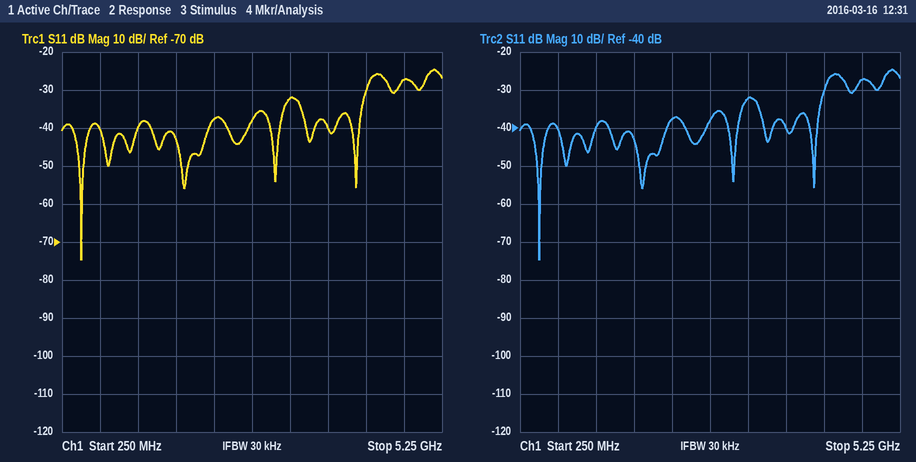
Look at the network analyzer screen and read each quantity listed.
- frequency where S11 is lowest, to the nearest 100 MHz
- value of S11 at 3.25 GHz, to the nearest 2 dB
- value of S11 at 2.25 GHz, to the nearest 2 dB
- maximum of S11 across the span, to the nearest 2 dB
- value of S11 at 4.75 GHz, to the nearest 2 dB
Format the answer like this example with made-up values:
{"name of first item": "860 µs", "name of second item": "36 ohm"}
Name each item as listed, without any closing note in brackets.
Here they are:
{"frequency where S11 is lowest, to the nearest 100 MHz": "500 MHz", "value of S11 at 3.25 GHz, to the nearest 2 dB": "-32 dB", "value of S11 at 2.25 GHz, to the nearest 2 dB": "-38 dB", "maximum of S11 across the span, to the nearest 2 dB": "-24 dB", "value of S11 at 4.75 GHz, to the nearest 2 dB": "-28 dB"}
